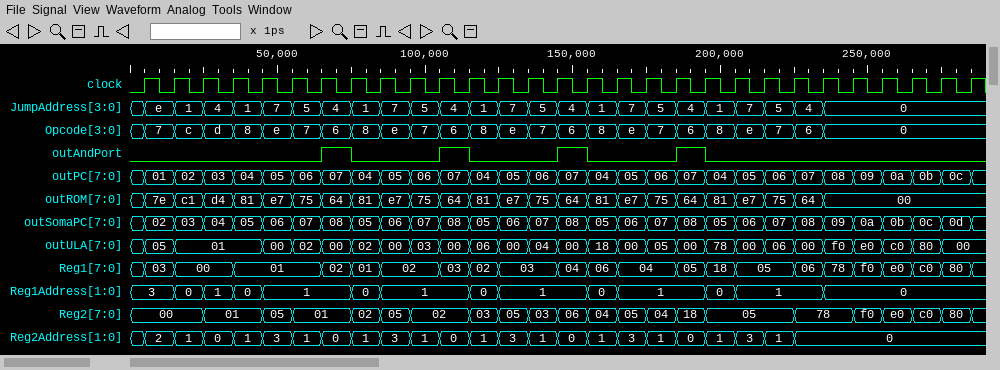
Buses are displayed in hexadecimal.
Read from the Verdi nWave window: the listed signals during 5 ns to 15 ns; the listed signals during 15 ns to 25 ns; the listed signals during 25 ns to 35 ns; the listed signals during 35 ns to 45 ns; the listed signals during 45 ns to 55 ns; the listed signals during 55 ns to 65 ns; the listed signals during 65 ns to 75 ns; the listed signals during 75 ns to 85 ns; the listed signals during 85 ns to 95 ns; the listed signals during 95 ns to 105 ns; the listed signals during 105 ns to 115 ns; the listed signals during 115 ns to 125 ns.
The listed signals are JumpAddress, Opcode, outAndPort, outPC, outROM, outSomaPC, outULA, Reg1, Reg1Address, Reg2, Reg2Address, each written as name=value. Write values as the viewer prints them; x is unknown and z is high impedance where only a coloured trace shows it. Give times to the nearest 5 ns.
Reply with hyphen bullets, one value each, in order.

- JumpAddress=e, Opcode=7, outAndPort=0, outPC=01, outROM=7e, outSomaPC=02, outULA=05, Reg1=03, Reg1Address=3, Reg2=00, Reg2Address=2
- JumpAddress=1, Opcode=c, outAndPort=0, outPC=02, outROM=c1, outSomaPC=03, outULA=01, Reg1=00, Reg1Address=0, Reg2=00, Reg2Address=1
- JumpAddress=4, Opcode=d, outAndPort=0, outPC=03, outROM=d4, outSomaPC=04, outULA=01, Reg1=00, Reg1Address=1, Reg2=01, Reg2Address=0
- JumpAddress=1, Opcode=8, outAndPort=0, outPC=04, outROM=81, outSomaPC=05, outULA=01, Reg1=01, Reg1Address=0, Reg2=01, Reg2Address=1
- JumpAddress=7, Opcode=e, outAndPort=0, outPC=05, outROM=e7, outSomaPC=06, outULA=00, Reg1=01, Reg1Address=1, Reg2=05, Reg2Address=3
- JumpAddress=5, Opcode=7, outAndPort=0, outPC=06, outROM=75, outSomaPC=07, outULA=02, Reg1=01, Reg1Address=1, Reg2=01, Reg2Address=1
- JumpAddress=4, Opcode=6, outAndPort=1, outPC=07, outROM=64, outSomaPC=08, outULA=00, Reg1=02, Reg1Address=1, Reg2=01, Reg2Address=0
- JumpAddress=1, Opcode=8, outAndPort=0, outPC=04, outROM=81, outSomaPC=05, outULA=02, Reg1=01, Reg1Address=0, Reg2=02, Reg2Address=1
- JumpAddress=7, Opcode=e, outAndPort=0, outPC=05, outROM=e7, outSomaPC=06, outULA=00, Reg1=02, Reg1Address=1, Reg2=05, Reg2Address=3
- JumpAddress=5, Opcode=7, outAndPort=0, outPC=06, outROM=75, outSomaPC=07, outULA=03, Reg1=02, Reg1Address=1, Reg2=02, Reg2Address=1
- JumpAddress=4, Opcode=6, outAndPort=1, outPC=07, outROM=64, outSomaPC=08, outULA=00, Reg1=03, Reg1Address=1, Reg2=02, Reg2Address=0
- JumpAddress=1, Opcode=8, outAndPort=0, outPC=04, outROM=81, outSomaPC=05, outULA=06, Reg1=02, Reg1Address=0, Reg2=03, Reg2Address=1
